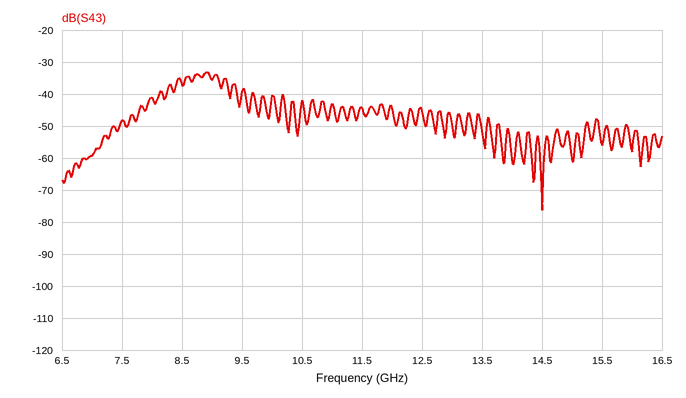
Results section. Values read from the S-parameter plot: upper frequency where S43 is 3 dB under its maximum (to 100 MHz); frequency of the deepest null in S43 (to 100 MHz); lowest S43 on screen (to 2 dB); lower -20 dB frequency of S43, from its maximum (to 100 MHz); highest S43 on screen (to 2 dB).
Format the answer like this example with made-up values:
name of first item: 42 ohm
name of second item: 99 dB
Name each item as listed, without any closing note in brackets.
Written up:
upper frequency where S43 is 3 dB under its maximum: 9.1 GHz
frequency of the deepest null in S43: 14.5 GHz
lowest S43 on screen: -76 dB
lower -20 dB frequency of S43, from its maximum: 7.3 GHz
highest S43 on screen: -34 dB
